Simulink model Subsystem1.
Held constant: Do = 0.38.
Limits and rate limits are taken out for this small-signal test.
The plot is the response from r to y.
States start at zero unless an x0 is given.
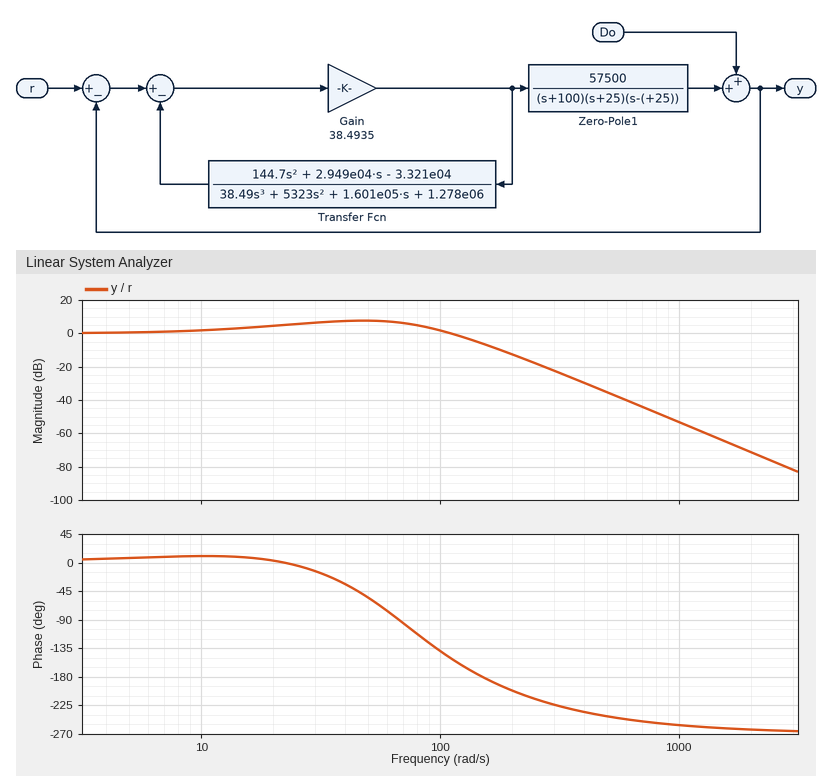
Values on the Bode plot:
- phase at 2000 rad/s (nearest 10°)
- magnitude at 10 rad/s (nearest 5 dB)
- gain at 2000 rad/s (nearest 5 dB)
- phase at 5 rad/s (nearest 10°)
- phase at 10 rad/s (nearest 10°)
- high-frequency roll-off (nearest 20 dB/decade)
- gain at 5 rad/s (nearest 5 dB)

-260°
0 dB
-70 dB
10°
10°
-60 dB/decade
0 dB
